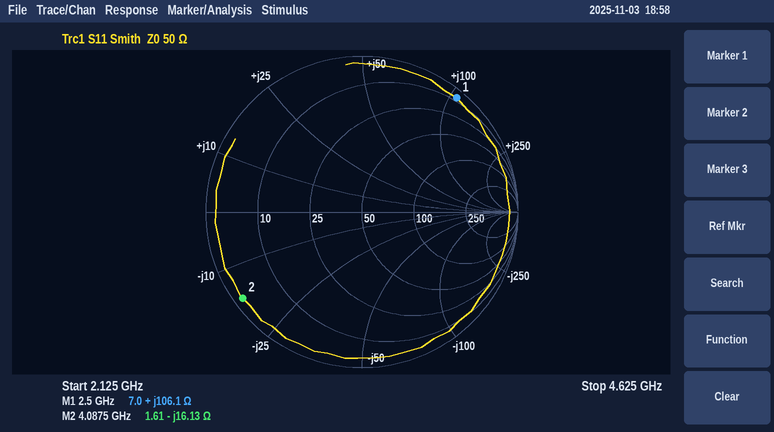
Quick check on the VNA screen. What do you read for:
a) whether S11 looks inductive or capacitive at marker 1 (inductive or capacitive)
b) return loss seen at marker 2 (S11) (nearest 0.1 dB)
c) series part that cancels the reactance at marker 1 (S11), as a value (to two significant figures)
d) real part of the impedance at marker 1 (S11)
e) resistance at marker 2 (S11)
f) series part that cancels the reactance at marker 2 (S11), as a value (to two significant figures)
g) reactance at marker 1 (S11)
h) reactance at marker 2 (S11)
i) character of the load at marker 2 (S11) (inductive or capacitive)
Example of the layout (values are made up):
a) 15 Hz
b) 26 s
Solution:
a) inductive
b) 0.5 dB
c) 600 fF
d) 7.0 Ω
e) 1.61 Ω
f) 630 pH
g) +106.1 Ω
h) -16.13 Ω
i) capacitive
